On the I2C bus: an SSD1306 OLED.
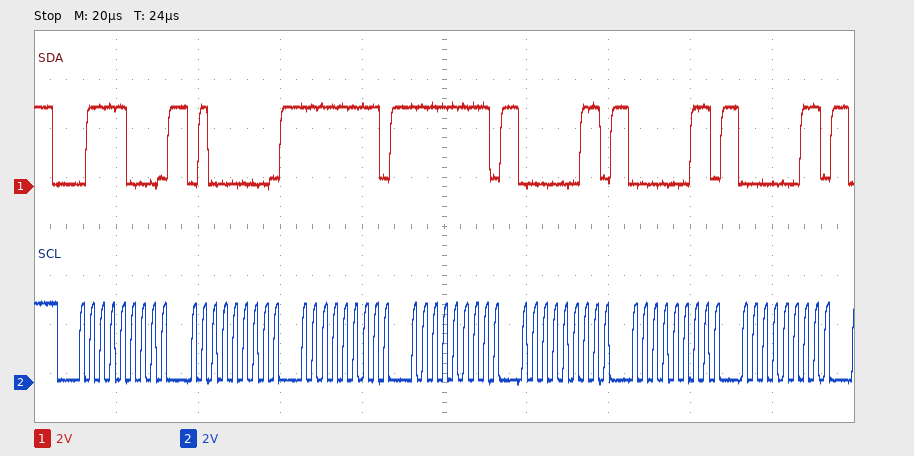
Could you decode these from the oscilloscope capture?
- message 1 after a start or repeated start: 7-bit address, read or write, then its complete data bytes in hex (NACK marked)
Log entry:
0x3C write: 40 FF FF 03 03 03
